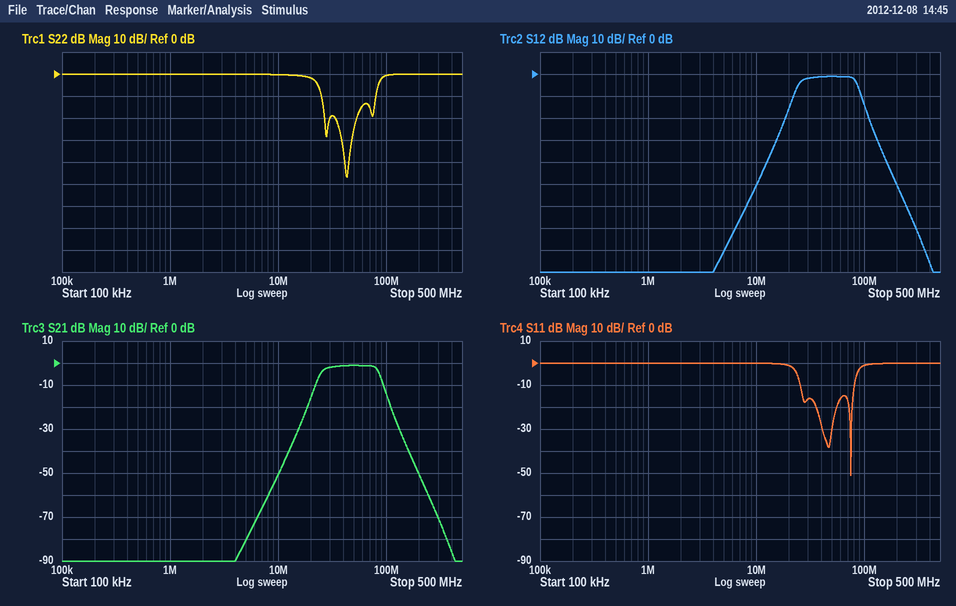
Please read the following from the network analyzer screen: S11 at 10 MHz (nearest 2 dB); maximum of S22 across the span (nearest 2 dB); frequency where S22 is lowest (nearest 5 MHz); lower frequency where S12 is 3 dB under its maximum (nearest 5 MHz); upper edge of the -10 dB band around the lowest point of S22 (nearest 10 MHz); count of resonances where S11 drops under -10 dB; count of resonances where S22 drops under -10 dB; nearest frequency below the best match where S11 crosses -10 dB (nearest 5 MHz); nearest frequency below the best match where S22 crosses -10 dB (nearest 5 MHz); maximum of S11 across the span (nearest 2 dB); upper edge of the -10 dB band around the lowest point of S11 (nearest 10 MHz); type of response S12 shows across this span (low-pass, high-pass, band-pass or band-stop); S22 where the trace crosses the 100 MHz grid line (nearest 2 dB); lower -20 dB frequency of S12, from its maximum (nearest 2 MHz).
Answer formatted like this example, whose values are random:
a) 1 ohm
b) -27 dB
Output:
a) 0 dB
b) 0 dB
c) 45 MHz
d) 25 MHz
e) 80 MHz
f) 2
g) 3
h) 25 MHz
i) 25 MHz
j) 0 dB
k) 80 MHz
l) band-pass
m) 0 dB
n) 18 MHz
